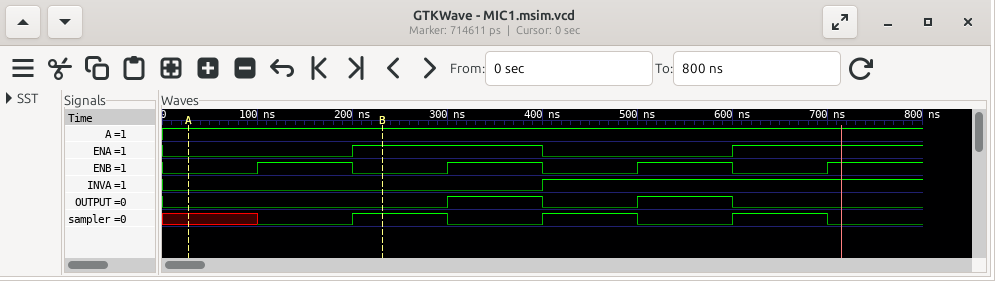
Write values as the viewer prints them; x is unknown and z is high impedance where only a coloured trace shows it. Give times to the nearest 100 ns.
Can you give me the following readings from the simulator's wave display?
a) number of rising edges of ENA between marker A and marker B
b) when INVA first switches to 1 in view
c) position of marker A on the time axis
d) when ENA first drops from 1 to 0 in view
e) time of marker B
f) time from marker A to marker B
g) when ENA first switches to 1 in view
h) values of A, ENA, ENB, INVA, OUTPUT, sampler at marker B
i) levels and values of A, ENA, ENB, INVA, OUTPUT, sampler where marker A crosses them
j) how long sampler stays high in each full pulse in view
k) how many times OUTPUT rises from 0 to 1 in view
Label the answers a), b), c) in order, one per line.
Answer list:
a) 1
b) 400 ns
c) 0 ns
d) 400 ns
e) 200 ns
f) 200 ns
g) 200 ns
h) A=1, ENA=1, ENB=0, INVA=0, OUTPUT=0, sampler=1
i) A=1, ENA=0, ENB=0, INVA=0, OUTPUT=0, sampler=x
j) 100 ns, 100 ns, 100 ns
k) 2
